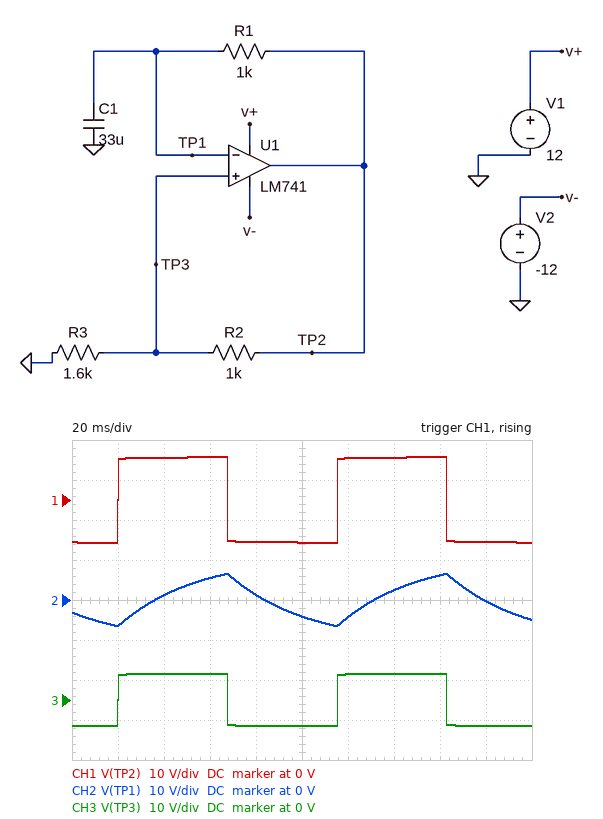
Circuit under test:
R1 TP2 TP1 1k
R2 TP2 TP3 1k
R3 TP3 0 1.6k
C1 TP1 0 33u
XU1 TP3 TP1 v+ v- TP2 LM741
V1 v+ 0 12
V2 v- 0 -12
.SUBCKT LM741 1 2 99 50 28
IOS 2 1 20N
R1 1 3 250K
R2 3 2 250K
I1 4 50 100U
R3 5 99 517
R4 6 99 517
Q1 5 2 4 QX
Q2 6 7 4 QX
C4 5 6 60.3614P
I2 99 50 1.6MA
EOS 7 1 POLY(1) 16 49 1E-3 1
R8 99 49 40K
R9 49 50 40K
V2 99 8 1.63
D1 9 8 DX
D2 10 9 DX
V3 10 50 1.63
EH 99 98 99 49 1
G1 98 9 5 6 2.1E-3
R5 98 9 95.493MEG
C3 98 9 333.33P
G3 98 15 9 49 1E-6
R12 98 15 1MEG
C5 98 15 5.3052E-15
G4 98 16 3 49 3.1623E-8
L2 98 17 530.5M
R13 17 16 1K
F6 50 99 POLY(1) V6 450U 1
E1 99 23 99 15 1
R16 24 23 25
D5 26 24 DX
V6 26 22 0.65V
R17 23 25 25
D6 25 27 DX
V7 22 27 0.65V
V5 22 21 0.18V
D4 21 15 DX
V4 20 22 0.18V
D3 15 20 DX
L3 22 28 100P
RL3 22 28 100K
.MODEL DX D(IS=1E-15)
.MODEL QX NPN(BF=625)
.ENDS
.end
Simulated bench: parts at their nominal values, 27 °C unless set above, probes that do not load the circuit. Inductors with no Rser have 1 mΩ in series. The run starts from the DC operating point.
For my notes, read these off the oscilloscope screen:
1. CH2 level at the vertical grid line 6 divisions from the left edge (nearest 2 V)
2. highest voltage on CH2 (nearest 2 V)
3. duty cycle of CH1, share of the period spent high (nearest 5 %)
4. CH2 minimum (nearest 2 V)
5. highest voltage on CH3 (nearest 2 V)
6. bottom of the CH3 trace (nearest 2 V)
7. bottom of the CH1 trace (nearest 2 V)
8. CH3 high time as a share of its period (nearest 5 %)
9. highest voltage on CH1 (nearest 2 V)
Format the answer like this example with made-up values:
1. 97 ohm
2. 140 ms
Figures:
1. -4 V
2. 6 V
3. 50 %
4. -6 V
5. 6 V
6. -6 V
7. -10 V
8. 50 %
9. 10 V
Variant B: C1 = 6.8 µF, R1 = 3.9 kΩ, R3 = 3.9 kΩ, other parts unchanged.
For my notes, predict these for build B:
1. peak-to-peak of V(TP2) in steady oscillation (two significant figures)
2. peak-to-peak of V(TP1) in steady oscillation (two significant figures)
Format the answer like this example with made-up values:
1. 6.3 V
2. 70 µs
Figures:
1. 22 V
2. 17 V
